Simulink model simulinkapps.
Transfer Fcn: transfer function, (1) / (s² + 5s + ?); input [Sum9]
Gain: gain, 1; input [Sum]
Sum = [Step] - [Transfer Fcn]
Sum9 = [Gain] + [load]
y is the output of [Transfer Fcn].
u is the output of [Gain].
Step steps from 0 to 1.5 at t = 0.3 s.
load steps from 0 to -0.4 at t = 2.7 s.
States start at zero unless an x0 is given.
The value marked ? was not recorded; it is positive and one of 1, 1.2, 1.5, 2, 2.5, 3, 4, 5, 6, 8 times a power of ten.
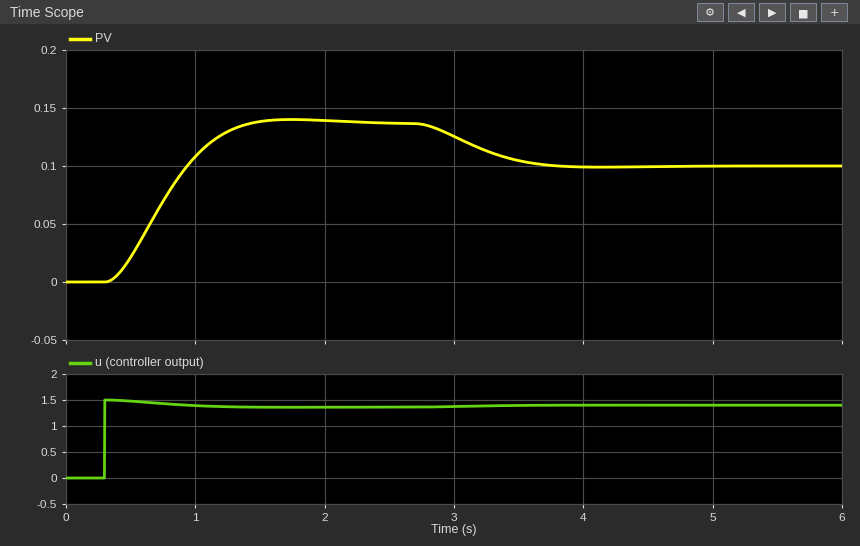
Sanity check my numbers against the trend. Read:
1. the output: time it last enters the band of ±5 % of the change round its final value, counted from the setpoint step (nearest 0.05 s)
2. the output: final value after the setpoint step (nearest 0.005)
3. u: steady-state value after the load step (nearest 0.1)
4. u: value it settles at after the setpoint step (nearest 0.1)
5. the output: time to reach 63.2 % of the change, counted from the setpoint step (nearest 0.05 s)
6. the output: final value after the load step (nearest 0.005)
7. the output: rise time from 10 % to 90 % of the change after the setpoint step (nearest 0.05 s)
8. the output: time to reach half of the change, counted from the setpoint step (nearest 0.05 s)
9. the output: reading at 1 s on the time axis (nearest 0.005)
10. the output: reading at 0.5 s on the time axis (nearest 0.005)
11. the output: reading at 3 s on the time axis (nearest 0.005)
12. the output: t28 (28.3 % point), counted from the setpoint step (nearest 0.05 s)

0.95 s
0.135
1.4
1.4
0.55 s
0.100
0.70 s
0.45 s
0.110
0.020
0.125
0.30 s
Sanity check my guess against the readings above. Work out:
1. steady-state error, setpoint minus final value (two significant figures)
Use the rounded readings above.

1.4
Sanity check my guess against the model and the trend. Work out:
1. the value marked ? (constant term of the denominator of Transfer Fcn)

10
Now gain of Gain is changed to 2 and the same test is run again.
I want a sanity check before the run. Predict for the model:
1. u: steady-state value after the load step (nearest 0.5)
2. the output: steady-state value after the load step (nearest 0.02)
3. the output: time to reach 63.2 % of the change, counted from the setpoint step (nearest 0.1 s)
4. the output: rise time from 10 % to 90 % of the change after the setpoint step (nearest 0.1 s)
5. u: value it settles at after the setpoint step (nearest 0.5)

2.5
0.22
0.5 s
0.6 s
2.5
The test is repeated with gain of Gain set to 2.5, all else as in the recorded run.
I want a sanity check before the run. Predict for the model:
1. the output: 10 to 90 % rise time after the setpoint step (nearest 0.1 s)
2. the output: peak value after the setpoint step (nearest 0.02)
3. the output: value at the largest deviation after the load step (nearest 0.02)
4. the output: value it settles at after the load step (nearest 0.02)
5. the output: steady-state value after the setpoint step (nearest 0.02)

0.6 s
0.32
0.26
0.26
0.30
